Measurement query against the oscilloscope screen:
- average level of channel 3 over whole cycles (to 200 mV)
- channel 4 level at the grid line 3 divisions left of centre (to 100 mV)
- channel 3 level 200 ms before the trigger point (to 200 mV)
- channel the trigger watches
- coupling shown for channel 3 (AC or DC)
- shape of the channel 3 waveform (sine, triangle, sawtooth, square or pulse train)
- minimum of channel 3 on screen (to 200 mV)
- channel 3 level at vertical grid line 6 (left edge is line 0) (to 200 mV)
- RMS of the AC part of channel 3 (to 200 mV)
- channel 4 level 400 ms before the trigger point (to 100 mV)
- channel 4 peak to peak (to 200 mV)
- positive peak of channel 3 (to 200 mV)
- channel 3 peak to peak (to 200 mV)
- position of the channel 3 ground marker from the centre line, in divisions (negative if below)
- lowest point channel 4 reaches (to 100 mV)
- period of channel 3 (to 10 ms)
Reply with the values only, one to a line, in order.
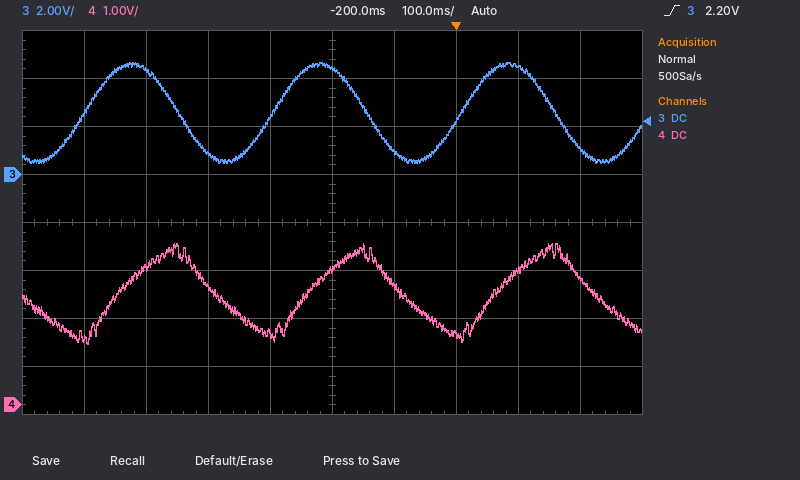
2.6 V
2.9 V
4.4 V
channel 3
DC
sine
400 mV
1.0 V
1.4 V
2.5 V
2.0 V
4.6 V
4.2 V
+1.0 div
1.3 V
300 ms
